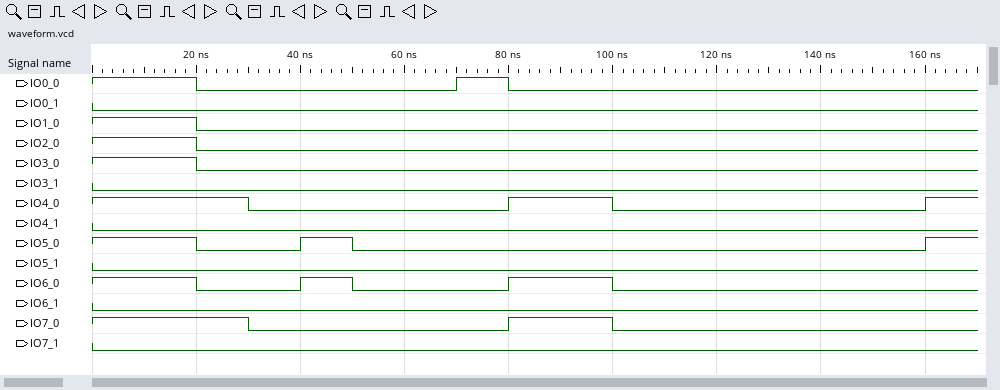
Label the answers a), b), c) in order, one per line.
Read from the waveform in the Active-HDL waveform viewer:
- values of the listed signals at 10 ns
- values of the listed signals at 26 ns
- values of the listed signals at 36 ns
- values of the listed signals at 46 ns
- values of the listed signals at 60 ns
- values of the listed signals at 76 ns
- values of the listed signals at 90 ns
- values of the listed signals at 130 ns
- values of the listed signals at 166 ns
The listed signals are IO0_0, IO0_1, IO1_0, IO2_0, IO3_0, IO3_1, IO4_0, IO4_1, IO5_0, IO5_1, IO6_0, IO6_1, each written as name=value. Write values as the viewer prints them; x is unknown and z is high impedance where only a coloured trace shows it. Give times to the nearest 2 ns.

a) IO0_0=1, IO0_1=0, IO1_0=1, IO2_0=1, IO3_0=1, IO3_1=0, IO4_0=1, IO4_1=0, IO5_0=1, IO5_1=0, IO6_0=1, IO6_1=0
b) IO0_0=0, IO0_1=0, IO1_0=0, IO2_0=0, IO3_0=0, IO3_1=0, IO4_0=1, IO4_1=0, IO5_0=0, IO5_1=0, IO6_0=0, IO6_1=0
c) IO0_0=0, IO0_1=0, IO1_0=0, IO2_0=0, IO3_0=0, IO3_1=0, IO4_0=0, IO4_1=0, IO5_0=0, IO5_1=0, IO6_0=0, IO6_1=0
d) IO0_0=0, IO0_1=0, IO1_0=0, IO2_0=0, IO3_0=0, IO3_1=0, IO4_0=0, IO4_1=0, IO5_0=1, IO5_1=0, IO6_0=1, IO6_1=0
e) IO0_0=0, IO0_1=0, IO1_0=0, IO2_0=0, IO3_0=0, IO3_1=0, IO4_0=0, IO4_1=0, IO5_0=0, IO5_1=0, IO6_0=0, IO6_1=0
f) IO0_0=1, IO0_1=0, IO1_0=0, IO2_0=0, IO3_0=0, IO3_1=0, IO4_0=0, IO4_1=0, IO5_0=0, IO5_1=0, IO6_0=0, IO6_1=0
g) IO0_0=0, IO0_1=0, IO1_0=0, IO2_0=0, IO3_0=0, IO3_1=0, IO4_0=1, IO4_1=0, IO5_0=0, IO5_1=0, IO6_0=1, IO6_1=0
h) IO0_0=0, IO0_1=0, IO1_0=0, IO2_0=0, IO3_0=0, IO3_1=0, IO4_0=0, IO4_1=0, IO5_0=0, IO5_1=0, IO6_0=0, IO6_1=0
i) IO0_0=0, IO0_1=0, IO1_0=0, IO2_0=0, IO3_0=0, IO3_1=0, IO4_0=1, IO4_1=0, IO5_0=1, IO5_1=0, IO6_0=0, IO6_1=0
